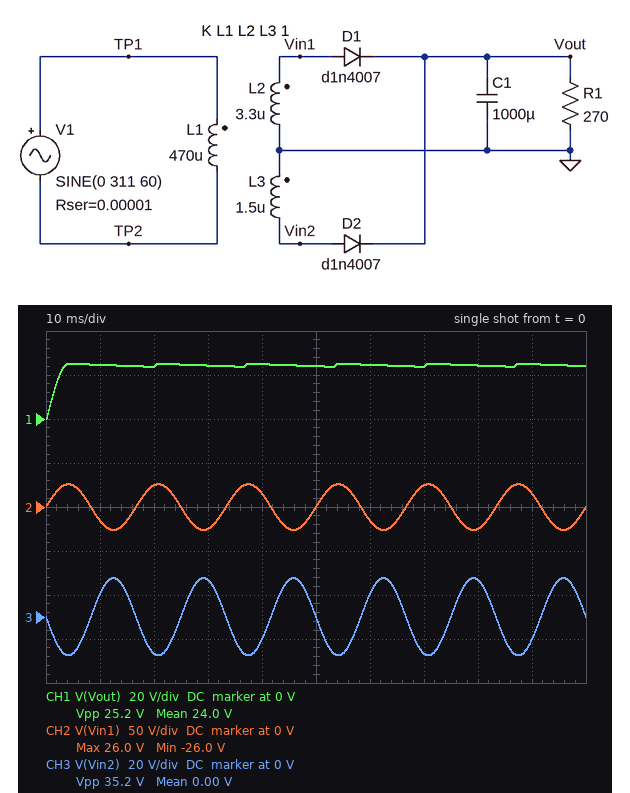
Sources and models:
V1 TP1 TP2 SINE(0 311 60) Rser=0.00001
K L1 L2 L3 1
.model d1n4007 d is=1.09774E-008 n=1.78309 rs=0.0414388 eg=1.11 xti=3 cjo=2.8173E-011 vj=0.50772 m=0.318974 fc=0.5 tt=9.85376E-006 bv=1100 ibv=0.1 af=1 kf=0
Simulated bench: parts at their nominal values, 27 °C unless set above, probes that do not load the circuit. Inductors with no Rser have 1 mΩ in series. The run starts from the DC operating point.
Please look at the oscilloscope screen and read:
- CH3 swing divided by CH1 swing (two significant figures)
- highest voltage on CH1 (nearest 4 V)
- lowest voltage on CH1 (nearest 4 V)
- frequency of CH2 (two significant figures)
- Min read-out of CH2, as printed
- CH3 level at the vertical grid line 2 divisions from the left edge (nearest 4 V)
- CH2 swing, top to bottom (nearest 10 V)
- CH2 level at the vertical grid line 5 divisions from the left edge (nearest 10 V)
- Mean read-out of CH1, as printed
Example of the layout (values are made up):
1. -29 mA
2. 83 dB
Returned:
1. 1.4
2. 24 V
3. 0 V
4. 60 Hz
5. -26.0 V
6. -16 V
7. 50 V
8. 0 V
9. 24.0 V
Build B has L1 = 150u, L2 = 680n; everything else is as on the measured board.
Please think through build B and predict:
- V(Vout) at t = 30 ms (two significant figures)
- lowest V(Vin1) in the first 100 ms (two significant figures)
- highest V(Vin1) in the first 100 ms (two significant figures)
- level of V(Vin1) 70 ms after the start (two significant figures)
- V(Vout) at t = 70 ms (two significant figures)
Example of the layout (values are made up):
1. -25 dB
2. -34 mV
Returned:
1. 31 V
2. -21 V
3. 21 V
4. 20 V
5. 30 V
